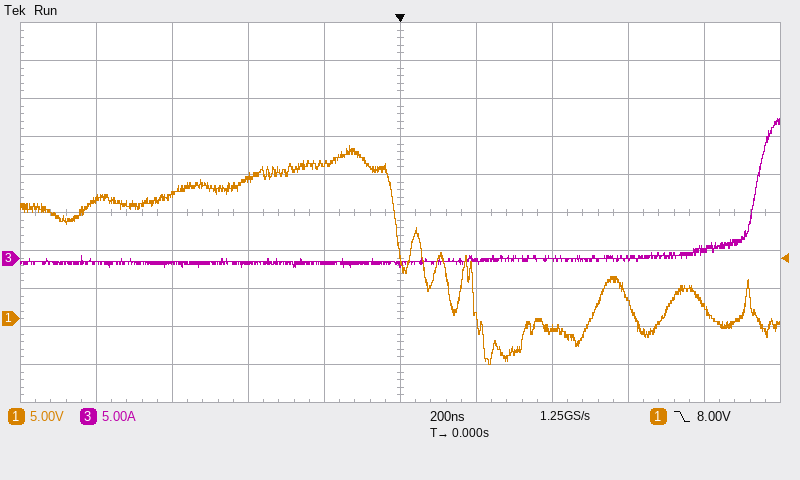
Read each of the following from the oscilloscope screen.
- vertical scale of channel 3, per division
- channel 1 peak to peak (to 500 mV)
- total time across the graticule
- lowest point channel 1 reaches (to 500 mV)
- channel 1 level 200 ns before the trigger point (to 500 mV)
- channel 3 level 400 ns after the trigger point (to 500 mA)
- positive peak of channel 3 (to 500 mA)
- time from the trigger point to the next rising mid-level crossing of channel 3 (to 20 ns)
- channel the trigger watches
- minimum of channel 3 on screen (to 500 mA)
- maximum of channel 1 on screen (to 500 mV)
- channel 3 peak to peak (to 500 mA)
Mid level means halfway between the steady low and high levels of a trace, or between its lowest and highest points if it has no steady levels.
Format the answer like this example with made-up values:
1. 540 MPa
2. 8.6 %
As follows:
1. 5 A
2. 29.0 V
3. 2 µs
4. -6.0 V
5. 20.5 V
6. 0.0 A
7. 18.5 A
8. 940 ns
9. channel 1
10. -1.0 A
11. 23.0 V
12. 19.5 A
